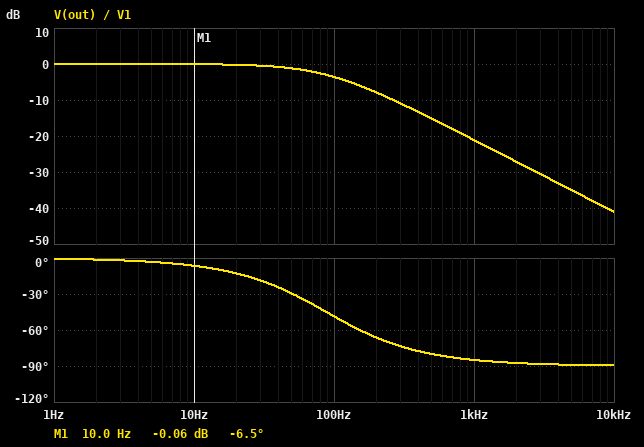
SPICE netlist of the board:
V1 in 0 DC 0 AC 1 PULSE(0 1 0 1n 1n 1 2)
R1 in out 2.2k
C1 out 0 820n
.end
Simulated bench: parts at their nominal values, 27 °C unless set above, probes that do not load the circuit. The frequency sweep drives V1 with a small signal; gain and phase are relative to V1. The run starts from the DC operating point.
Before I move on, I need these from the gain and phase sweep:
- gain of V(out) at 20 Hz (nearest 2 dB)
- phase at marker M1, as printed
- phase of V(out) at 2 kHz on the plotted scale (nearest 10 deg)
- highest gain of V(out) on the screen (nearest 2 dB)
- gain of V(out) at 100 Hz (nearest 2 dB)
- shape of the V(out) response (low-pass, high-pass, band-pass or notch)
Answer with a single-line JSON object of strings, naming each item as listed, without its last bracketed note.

{"gain of V(out) at 20 Hz": "0 dB", "phase at marker M1, as printed": "-6.5 deg", "phase of V(out) at 2 kHz on the plotted scale": "-90 deg", "highest gain of V(out) on the screen": "0 dB", "gain of V(out) at 100 Hz": "-4 dB", "shape of the V(out) response": "low-pass"}
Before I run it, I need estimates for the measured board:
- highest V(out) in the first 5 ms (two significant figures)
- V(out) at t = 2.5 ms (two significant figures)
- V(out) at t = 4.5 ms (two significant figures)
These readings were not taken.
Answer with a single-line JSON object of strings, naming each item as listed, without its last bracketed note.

{"highest V(out) in the first 5 ms": "940 mV", "V(out) at t = 2.5 ms": "750 mV", "V(out) at t = 4.5 ms": "920 mV"}
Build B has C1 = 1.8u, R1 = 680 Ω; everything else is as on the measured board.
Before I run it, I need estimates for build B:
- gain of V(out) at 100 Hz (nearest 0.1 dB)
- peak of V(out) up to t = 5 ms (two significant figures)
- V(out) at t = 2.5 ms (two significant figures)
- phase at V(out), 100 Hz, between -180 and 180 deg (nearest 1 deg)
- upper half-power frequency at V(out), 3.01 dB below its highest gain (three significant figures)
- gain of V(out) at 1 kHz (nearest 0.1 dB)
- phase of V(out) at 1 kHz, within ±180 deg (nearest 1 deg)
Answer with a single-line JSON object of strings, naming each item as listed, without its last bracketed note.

{"gain of V(out) at 100 Hz": "-2.0 dB", "peak of V(out) up to t = 5 ms": "980 mV", "V(out) at t = 2.5 ms": "870 mV", "phase at V(out), 100 Hz, between -180 and 180 deg": "-38 deg", "upper half-power frequency at V(out), 3.01 dB below its highest gain": "130 Hz", "gain of V(out) at 1 kHz": "-17.8 dB", "phase of V(out) at 1 kHz, within ±180 deg": "-83 deg"}
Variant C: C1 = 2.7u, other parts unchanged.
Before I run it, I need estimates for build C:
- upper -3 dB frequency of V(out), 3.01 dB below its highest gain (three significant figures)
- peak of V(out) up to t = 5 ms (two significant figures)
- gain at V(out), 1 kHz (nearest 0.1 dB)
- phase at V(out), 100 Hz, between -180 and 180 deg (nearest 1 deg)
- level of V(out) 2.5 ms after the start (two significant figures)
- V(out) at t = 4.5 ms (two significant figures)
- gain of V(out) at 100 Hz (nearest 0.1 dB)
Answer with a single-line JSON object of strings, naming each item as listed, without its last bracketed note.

{"upper -3 dB frequency of V(out), 3.01 dB below its highest gain": "26.8 Hz", "peak of V(out) up to t = 5 ms": "570 mV", "gain at V(out), 1 kHz": "-31.4 dB", "phase at V(out), 100 Hz, between -180 and 180 deg": "-75 deg", "level of V(out) 2.5 ms after the start": "340 mV", "V(out) at t = 4.5 ms": "530 mV", "gain of V(out) at 100 Hz": "-11.7 dB"}
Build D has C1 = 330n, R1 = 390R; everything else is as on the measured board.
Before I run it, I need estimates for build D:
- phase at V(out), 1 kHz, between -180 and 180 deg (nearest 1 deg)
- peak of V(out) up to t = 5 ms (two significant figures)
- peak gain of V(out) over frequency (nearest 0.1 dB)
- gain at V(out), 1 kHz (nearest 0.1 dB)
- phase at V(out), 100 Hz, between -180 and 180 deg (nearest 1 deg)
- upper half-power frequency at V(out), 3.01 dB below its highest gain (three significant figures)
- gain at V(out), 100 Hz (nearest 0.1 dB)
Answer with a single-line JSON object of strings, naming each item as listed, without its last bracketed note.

{"phase at V(out), 1 kHz, between -180 and 180 deg": "-39 deg", "peak of V(out) up to t = 5 ms": "1.0 V", "peak gain of V(out) over frequency": "0 dB", "gain at V(out), 1 kHz": "-2.2 dB", "phase at V(out), 100 Hz, between -180 and 180 deg": "-5 deg", "upper half-power frequency at V(out), 3.01 dB below its highest gain": "1.24 kHz", "gain at V(out), 100 Hz": "0 dB"}
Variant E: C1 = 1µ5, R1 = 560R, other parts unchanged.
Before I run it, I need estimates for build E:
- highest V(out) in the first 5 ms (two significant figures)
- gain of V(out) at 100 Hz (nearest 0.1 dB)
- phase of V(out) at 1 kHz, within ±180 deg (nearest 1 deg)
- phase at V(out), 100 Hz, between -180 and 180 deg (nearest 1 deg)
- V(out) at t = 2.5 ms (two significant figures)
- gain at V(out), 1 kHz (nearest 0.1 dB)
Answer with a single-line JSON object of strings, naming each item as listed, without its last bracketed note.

{"highest V(out) in the first 5 ms": "1.0 V", "gain of V(out) at 100 Hz": "-1.1 dB", "phase of V(out) at 1 kHz, within ±180 deg": "-79 deg", "phase at V(out), 100 Hz, between -180 and 180 deg": "-28 deg", "V(out) at t = 2.5 ms": "950 mV", "gain at V(out), 1 kHz": "-14.6 dB"}
